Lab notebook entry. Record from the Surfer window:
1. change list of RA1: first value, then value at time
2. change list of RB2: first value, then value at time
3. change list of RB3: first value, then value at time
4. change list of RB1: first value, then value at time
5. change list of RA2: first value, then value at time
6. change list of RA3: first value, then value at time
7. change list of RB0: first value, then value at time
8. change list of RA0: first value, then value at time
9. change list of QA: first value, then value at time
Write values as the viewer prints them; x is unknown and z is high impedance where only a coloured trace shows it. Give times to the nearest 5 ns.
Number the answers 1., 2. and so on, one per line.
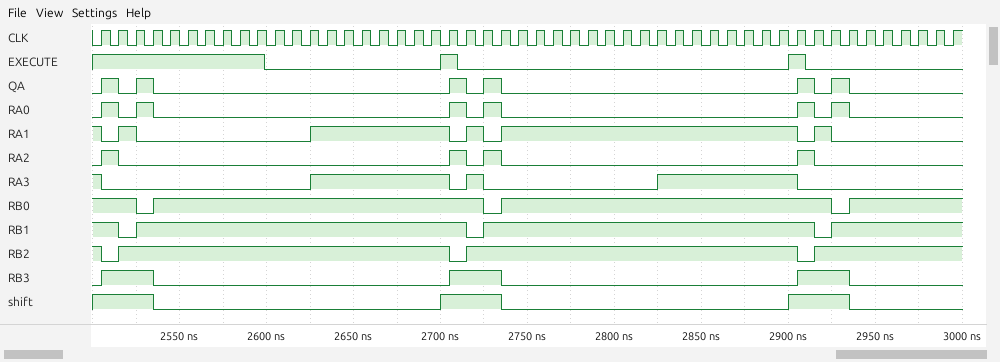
1. 1, 0 at 2505 ns, 1 at 2515 ns, 0 at 2525 ns, 1 at 2625 ns, 0 at 2705 ns, 1 at 2715 ns, 0 at 2725 ns, 1 at 2735 ns, 0 at 2905 ns, 1 at 2915 ns, 0 at 2925 ns
2. 1, 0 at 2505 ns, 1 at 2515 ns, 0 at 2705 ns, 1 at 2715 ns, 0 at 2905 ns, 1 at 2915 ns
3. 0, 1 at 2505 ns, 0 at 2535 ns, 1 at 2705 ns, 0 at 2735 ns, 1 at 2905 ns, 0 at 2935 ns
4. 1, 0 at 2515 ns, 1 at 2525 ns, 0 at 2715 ns, 1 at 2725 ns, 0 at 2915 ns, 1 at 2925 ns
5. 0, 1 at 2505 ns, 0 at 2515 ns, 1 at 2705 ns, 0 at 2715 ns, 1 at 2725 ns, 0 at 2735 ns, 1 at 2905 ns, 0 at 2915 ns
6. 1, 0 at 2505 ns, 1 at 2625 ns, 0 at 2705 ns, 1 at 2715 ns, 0 at 2725 ns, 1 at 2825 ns, 0 at 2905 ns
7. 1, 0 at 2525 ns, 1 at 2535 ns, 0 at 2725 ns, 1 at 2735 ns, 0 at 2925 ns, 1 at 2935 ns
8. 0, 1 at 2505 ns, 0 at 2515 ns, 1 at 2525 ns, 0 at 2535 ns, 1 at 2705 ns, 0 at 2715 ns, 1 at 2725 ns, 0 at 2735 ns, 1 at 2905 ns, 0 at 2915 ns, 1 at 2925 ns, 0 at 2935 ns
9. 0, 1 at 2505 ns, 0 at 2515 ns, 1 at 2525 ns, 0 at 2535 ns, 1 at 2705 ns, 0 at 2715 ns, 1 at 2725 ns, 0 at 2735 ns, 1 at 2905 ns, 0 at 2915 ns, 1 at 2925 ns, 0 at 2935 ns
